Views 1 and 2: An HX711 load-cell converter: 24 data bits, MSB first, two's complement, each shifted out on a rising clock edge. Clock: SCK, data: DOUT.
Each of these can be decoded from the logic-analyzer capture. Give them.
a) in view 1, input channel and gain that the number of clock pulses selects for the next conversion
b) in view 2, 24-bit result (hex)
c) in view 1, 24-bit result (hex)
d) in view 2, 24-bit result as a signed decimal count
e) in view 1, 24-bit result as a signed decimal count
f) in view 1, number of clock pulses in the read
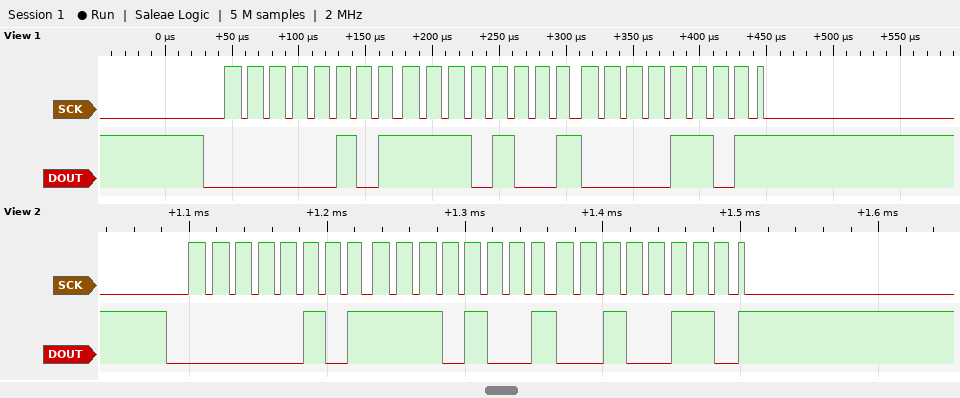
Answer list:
channel A, gain 128
0x05E926
0x05E90D
387366
387341
25
